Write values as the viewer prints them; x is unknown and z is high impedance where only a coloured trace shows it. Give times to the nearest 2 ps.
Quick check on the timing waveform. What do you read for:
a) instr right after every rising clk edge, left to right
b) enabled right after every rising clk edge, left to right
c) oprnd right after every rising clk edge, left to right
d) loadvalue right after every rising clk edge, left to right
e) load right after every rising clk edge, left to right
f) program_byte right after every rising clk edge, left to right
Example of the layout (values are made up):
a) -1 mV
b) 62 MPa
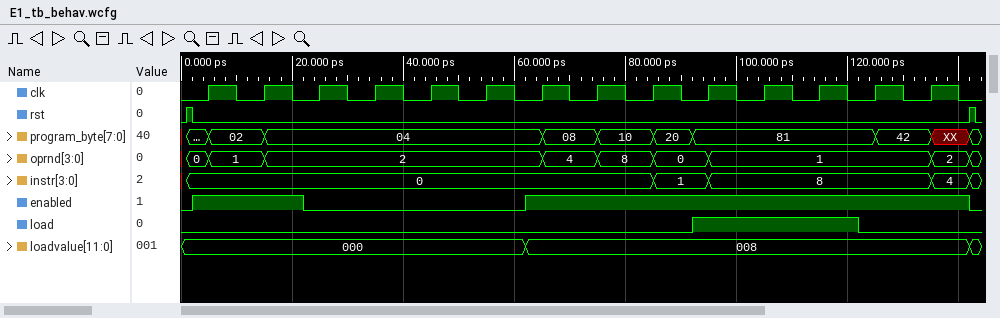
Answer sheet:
a) 0, 0, 0, 0, 0, 0, 0, 0, 1, 8, 8, 8, 8, 4
b) 1 1 0 0 0 0 1 1 1 1 1 1 1 1
c) 1, 2, 2, 2, 2, 2, 4, 8, 0, 1, 1, 1, 1, 2
d) 000, 000, 000, 000, 000, 000, 008, 008, 008, 008, 008, 008, 008, 008
e) 0 0 0 0 0 0 0 0 0 1 1 1 0 0
f) 02, 04, 04, 04, 04, 04, 08, 10, 20, 81, 81, 81, 42, XX
